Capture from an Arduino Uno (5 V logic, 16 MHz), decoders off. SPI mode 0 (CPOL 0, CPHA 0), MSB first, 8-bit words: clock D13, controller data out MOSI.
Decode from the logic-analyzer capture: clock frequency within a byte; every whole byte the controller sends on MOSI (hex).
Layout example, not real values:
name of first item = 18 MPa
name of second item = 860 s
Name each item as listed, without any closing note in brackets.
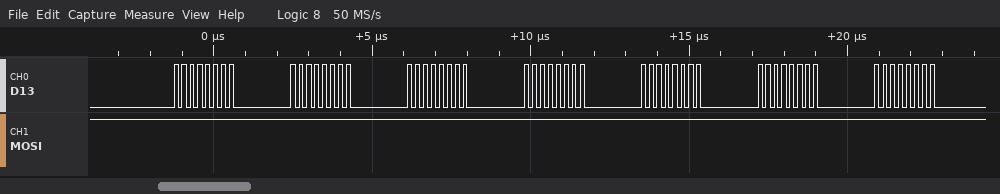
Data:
clock frequency within a byte = 4 MHz
every whole byte the controller sends on MOSI = FF FF FF FF FF FF FF
